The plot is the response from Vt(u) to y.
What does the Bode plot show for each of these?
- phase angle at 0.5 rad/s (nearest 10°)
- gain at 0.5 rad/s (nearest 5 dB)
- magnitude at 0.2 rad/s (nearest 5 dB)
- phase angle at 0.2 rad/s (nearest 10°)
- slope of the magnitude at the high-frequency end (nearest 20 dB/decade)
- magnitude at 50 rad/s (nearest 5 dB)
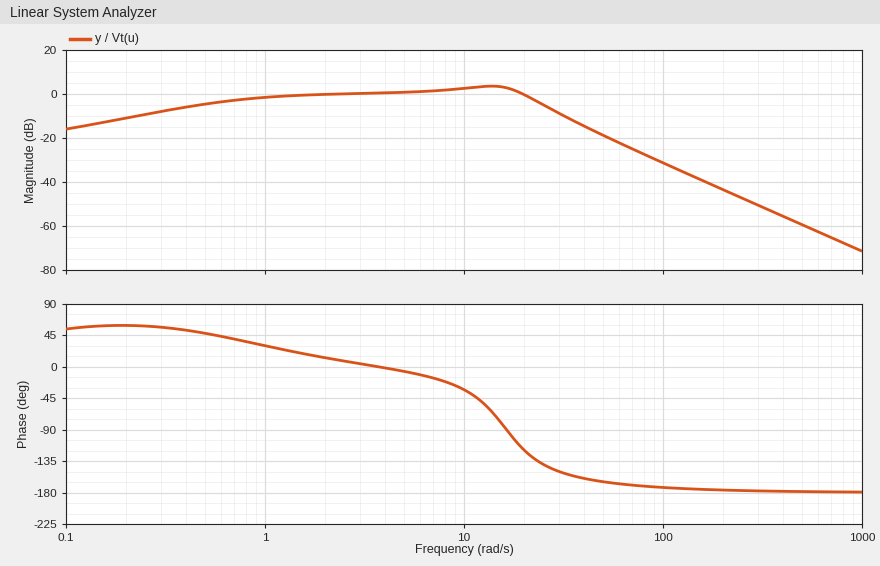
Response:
50°
-5 dB
-10 dB
60°
-40 dB/decade
-20 dB
